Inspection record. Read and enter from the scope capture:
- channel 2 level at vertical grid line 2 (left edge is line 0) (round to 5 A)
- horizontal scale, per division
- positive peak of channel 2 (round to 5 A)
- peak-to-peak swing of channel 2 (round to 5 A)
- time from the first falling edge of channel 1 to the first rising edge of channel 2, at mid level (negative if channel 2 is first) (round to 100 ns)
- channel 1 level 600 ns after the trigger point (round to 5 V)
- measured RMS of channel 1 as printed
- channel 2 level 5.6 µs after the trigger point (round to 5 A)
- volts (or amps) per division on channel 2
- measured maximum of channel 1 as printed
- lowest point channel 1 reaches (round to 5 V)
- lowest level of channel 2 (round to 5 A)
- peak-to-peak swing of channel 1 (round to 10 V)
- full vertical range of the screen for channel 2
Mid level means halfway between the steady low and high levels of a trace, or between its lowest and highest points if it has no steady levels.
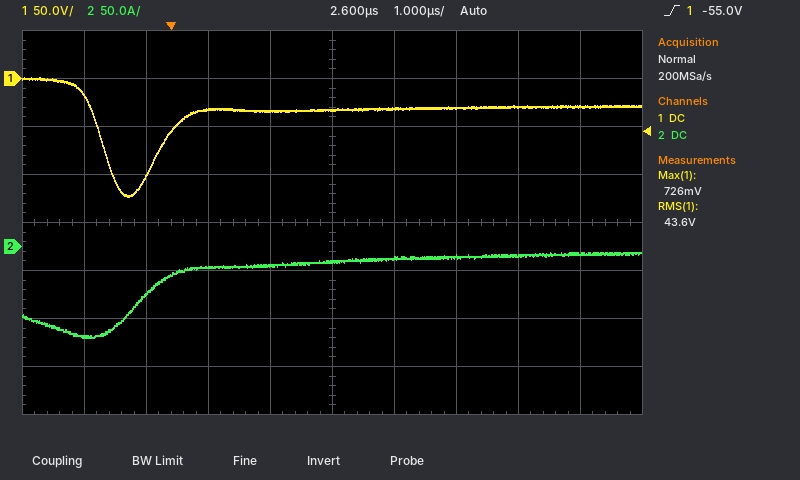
-50 A
1 µs
-5 A
90 A
+700 ns
-30 V
43.6 V
-10 A
50 A
726 mV
-125 V
-95 A
120 V
400 A
